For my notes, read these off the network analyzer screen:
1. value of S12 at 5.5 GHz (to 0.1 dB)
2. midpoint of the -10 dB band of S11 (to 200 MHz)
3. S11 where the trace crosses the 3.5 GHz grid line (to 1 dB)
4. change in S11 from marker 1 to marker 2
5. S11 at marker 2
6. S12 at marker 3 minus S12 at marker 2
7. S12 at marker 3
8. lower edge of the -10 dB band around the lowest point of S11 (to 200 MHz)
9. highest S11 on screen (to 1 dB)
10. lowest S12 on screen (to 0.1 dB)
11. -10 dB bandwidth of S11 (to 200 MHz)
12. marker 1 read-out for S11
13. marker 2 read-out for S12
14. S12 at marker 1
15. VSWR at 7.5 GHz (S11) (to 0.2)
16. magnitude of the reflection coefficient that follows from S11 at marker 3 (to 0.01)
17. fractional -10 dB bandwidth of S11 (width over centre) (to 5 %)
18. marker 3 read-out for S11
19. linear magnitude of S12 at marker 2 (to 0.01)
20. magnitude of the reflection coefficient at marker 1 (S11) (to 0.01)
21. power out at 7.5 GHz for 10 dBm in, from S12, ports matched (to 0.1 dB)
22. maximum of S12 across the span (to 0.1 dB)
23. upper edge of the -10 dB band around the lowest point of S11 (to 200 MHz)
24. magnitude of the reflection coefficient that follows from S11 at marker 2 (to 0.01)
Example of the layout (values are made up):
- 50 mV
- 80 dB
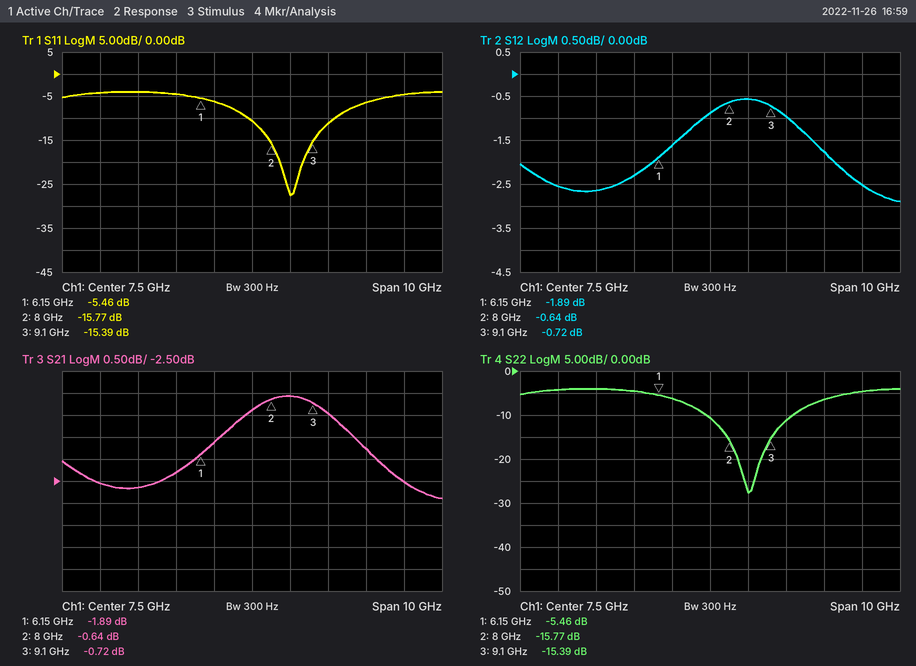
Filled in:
- -2.3 dB
- 8.6 GHz
- -4 dB
- -10.31 dB
- -15.77 dB
- -0.08 dB
- -0.72 dB
- 7.4 GHz
- -4 dB
- -2.9 dB
- 2.2 GHz
- -5.46 dB
- -0.64 dB
- -1.89 dB
- 1.8
- 0.17
- 25 %
- -15.39 dB
- 0.93
- 0.53
- 9.1 dBm
- -0.6 dB
- 9.6 GHz
- 0.16
